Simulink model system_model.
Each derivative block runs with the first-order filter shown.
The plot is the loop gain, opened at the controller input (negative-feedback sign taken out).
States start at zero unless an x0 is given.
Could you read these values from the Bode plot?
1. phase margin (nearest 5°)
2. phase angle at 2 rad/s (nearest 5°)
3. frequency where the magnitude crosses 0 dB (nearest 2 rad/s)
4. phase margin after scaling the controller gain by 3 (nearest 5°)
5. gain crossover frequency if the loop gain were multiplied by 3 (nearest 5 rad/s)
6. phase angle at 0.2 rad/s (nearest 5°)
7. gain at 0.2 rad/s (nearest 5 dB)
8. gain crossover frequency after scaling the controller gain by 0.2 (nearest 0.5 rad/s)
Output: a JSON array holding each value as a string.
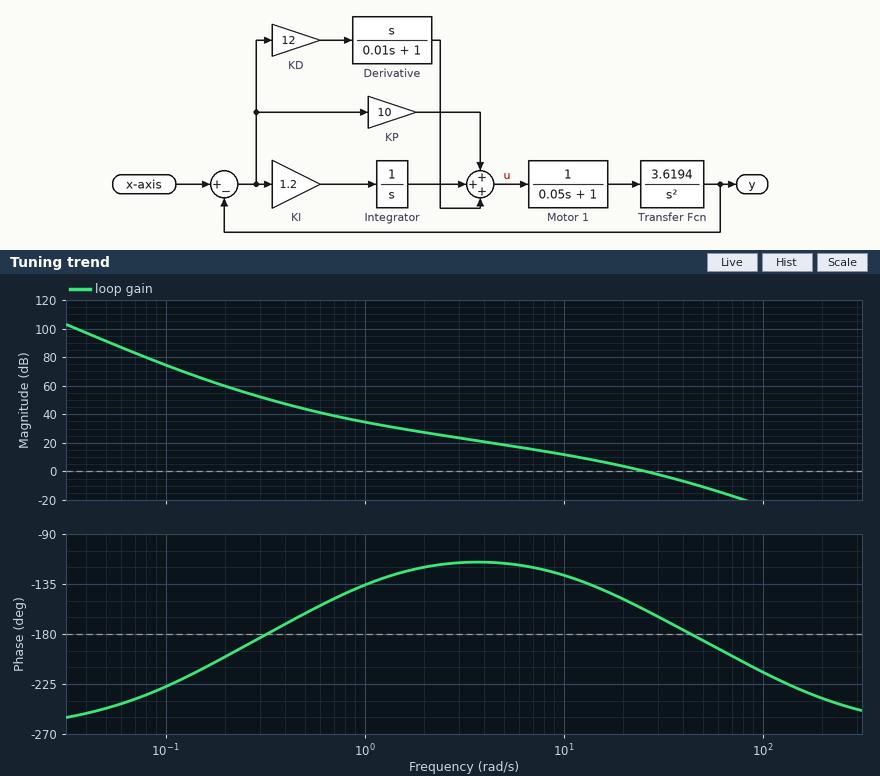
["20°", "-120°", "26 rad/s", "-5°", "45 rad/s", "-200°", "60 dB", "8.0 rad/s"]
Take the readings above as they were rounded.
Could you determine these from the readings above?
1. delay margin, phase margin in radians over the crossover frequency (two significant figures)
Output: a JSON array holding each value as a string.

["0.013 s"]
